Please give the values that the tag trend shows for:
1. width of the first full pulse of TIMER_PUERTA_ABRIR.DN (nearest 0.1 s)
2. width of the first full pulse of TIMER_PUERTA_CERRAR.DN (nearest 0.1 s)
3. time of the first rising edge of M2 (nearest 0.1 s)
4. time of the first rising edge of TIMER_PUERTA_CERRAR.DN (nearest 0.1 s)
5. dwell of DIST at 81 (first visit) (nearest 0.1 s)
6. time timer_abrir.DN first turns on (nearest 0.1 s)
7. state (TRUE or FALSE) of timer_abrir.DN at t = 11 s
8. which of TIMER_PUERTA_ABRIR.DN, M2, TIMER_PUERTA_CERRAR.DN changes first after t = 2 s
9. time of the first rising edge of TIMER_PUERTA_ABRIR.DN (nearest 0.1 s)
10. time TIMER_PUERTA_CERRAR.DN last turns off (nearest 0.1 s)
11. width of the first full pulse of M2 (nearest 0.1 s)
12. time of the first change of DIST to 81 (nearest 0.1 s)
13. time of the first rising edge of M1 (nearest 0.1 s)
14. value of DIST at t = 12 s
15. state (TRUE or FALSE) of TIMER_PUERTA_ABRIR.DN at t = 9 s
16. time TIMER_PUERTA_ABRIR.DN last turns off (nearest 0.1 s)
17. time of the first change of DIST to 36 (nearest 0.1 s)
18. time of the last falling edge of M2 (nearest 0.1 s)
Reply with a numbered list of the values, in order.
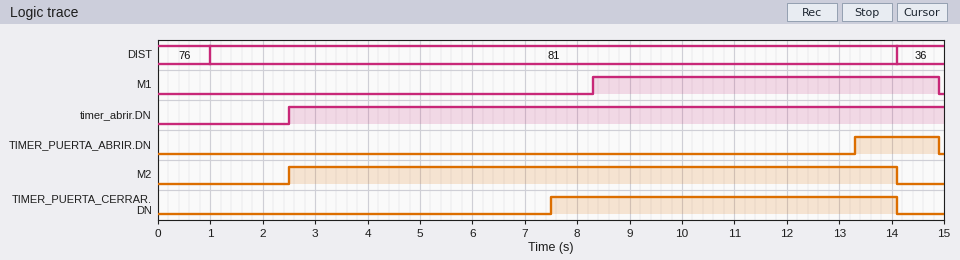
1. 1.6 s
2. 6.6 s
3. 2.5 s
4. 7.5 s
5. 13.1 s
6. 2.5 s
7. TRUE
8. M2
9. 13.3 s
10. 14.1 s
11. 11.6 s
12. 1.0 s
13. 8.3 s
14. 81
15. FALSE
16. 14.9 s
17. 14.1 s
18. 14.1 s
